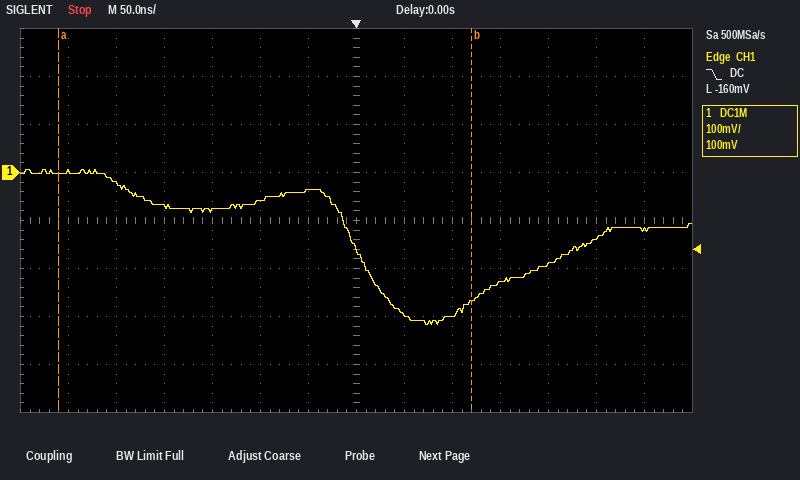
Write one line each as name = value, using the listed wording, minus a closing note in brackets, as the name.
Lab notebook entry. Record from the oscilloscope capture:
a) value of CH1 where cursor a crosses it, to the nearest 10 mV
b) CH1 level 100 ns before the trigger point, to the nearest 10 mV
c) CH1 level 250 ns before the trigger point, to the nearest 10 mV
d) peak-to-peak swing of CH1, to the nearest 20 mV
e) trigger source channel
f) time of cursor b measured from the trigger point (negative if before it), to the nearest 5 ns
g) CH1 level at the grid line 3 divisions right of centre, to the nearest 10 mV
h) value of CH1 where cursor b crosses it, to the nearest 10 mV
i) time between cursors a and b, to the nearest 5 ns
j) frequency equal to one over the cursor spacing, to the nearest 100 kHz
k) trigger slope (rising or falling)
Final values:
value of CH1 where cursor a crosses it, to the nearest 10 mV = 0 mV
CH1 level 100 ns before the trigger point, to the nearest 10 mV = -60 mV
CH1 level 250 ns before the trigger point, to the nearest 10 mV = -20 mV
peak-to-peak swing of CH1, to the nearest 20 mV = 320 mV
trigger source channel = CH1
time of cursor b measured from the trigger point (negative if before it), to the nearest 5 ns = +120 ns
CH1 level at the grid line 3 divisions right of centre, to the nearest 10 mV = -230 mV
value of CH1 where cursor b crosses it, to the nearest 10 mV = -270 mV
time between cursors a and b, to the nearest 5 ns = 430 ns
frequency equal to one over the cursor spacing, to the nearest 100 kHz = 2.3 MHz
trigger slope = falling
